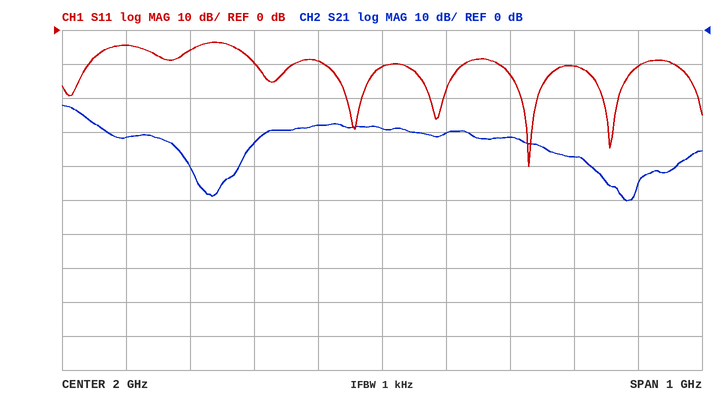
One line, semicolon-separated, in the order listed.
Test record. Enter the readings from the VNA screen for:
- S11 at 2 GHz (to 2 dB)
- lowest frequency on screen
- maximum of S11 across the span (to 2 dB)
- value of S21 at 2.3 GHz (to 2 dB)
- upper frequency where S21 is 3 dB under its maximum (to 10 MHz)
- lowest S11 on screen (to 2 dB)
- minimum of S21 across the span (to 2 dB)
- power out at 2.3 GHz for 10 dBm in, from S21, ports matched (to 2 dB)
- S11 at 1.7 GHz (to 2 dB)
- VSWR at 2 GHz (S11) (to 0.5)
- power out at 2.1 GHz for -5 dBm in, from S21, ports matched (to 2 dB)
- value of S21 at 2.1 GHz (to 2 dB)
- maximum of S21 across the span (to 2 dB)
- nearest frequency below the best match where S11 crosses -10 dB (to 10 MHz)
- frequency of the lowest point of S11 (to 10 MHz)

-10 dB; 1.5 GHz; -4 dB; -38 dB; 1.53 GHz; -40 dB; -50 dB; -28 dBm; -6 dB; 2.0; -36 dBm; -30 dB; -22 dB; 2.18 GHz; 2.23 GHz
